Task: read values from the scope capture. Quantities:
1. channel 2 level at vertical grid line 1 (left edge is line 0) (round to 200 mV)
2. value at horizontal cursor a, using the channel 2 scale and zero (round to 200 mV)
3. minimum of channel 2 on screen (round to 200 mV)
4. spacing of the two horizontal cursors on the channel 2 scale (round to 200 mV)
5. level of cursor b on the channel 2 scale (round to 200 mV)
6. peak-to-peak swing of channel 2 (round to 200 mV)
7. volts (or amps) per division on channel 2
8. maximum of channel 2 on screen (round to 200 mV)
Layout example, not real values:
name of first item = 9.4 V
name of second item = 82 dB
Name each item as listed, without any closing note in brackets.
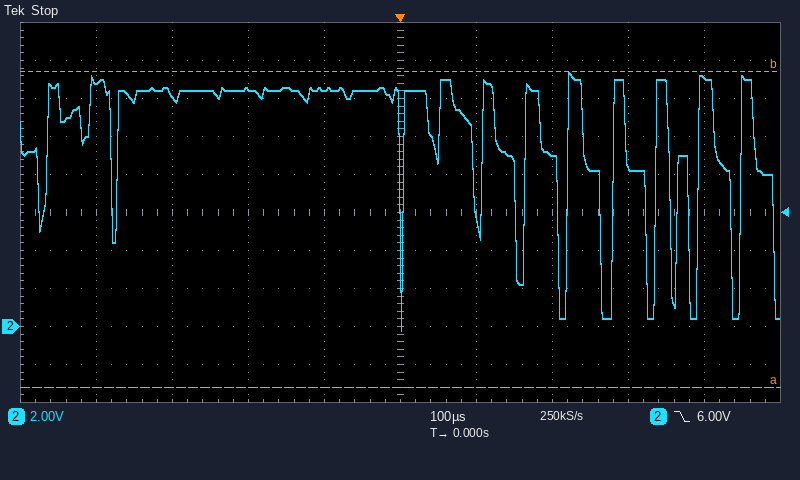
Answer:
channel 2 level at vertical grid line 1 (left edge is line 0) = 13.0 V
value at horizontal cursor a, using the channel 2 scale and zero = -3.2 V
minimum of channel 2 on screen = -200 mV
spacing of the two horizontal cursors on the channel 2 scale = 16.6 V
level of cursor b on the channel 2 scale = 13.4 V
peak-to-peak swing of channel 2 = 13.6 V
volts (or amps) per division on channel 2 = 2 V
maximum of channel 2 on screen = 13.4 V
